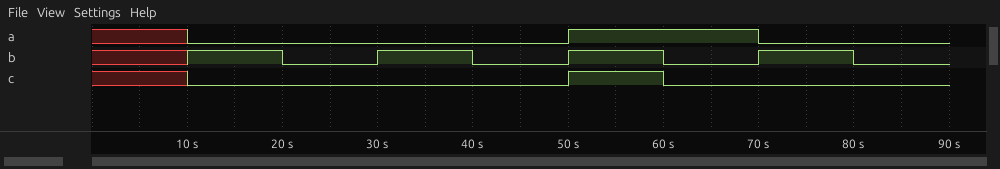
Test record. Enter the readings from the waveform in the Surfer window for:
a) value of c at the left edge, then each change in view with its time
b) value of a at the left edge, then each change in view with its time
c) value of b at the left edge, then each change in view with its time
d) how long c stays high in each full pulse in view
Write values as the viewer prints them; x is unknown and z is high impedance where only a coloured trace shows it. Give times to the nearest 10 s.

x, 0 at 10 s, 1 at 50 s, 0 at 60 s
x, 0 at 10 s, 1 at 50 s, 0 at 70 s
x, 1 at 10 s, 0 at 20 s, 1 at 30 s, 0 at 40 s, 1 at 50 s, 0 at 60 s, 1 at 70 s, 0 at 80 s
10 s
